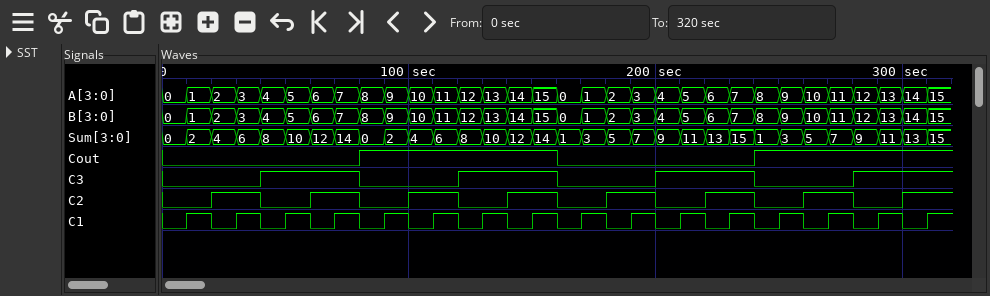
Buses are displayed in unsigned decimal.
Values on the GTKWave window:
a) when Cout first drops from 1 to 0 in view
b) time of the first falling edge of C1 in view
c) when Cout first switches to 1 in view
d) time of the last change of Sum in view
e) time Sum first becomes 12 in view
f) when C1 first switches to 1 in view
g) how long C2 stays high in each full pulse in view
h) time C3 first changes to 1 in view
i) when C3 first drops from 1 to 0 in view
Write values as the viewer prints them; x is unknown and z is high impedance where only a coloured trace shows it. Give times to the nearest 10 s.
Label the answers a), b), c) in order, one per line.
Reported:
a) 160 s
b) 20 s
c) 80 s
d) 310 s
e) 60 s
f) 10 s
g) 20 s, 20 s, 20 s, 20 s, 20 s, 20 s, 20 s
h) 40 s
i) 80 s
